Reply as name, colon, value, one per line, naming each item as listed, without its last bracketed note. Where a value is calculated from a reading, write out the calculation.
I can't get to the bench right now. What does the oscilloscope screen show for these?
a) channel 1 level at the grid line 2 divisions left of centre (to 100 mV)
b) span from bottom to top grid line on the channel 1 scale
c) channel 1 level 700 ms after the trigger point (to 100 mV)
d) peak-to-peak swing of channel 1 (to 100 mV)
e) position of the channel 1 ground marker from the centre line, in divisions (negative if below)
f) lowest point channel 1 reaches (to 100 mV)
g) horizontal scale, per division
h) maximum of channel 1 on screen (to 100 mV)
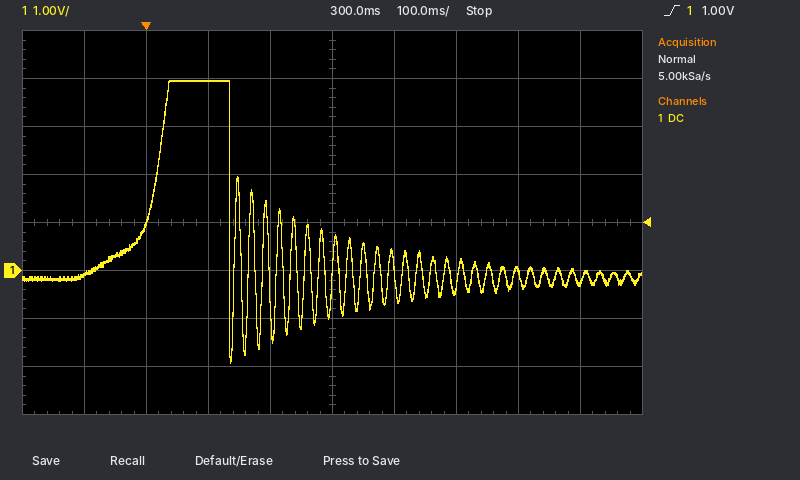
channel 1 level at the grid line 2 divisions left of centre: 4.0 V
span from bottom to top grid line on the channel 1 scale: 8 V
channel 1 level 700 ms after the trigger point: -200 mV
peak-to-peak swing of channel 1: 4.0 V − (-1.9 V) = 5.9 V
position of the channel 1 ground marker from the centre line, in divisions: -1.0 div
lowest point channel 1 reaches: -1.9 V
horizontal scale, per division: 100 ms
maximum of channel 1 on screen: 4.0 V
